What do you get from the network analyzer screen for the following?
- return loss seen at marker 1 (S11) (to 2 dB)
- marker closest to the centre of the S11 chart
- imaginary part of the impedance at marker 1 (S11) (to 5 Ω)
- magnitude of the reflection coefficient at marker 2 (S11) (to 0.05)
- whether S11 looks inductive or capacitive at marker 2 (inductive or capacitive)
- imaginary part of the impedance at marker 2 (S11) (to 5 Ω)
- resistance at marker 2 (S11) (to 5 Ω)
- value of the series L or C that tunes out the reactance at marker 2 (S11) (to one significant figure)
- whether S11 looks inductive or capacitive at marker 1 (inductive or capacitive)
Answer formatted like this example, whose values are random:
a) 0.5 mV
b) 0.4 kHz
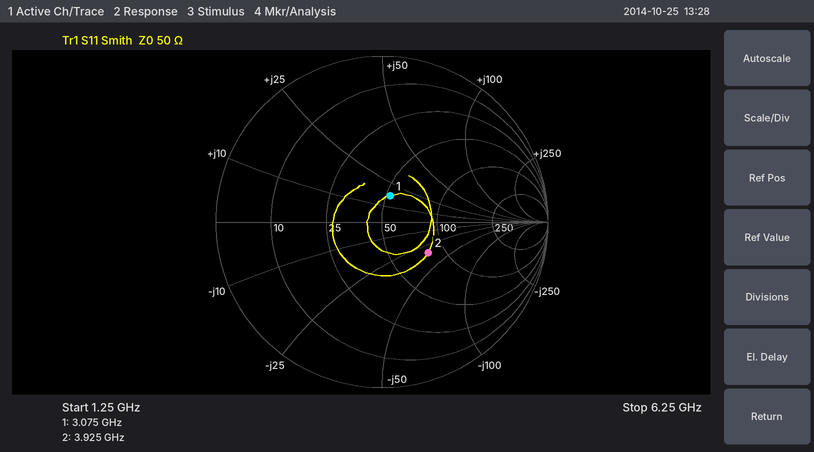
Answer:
a) 16 dB
b) marker 1
c) +15 Ω
d) 0.35
e) capacitive
f) -35 Ω
g) 80 Ω
h) 1 nH
i) inductive
